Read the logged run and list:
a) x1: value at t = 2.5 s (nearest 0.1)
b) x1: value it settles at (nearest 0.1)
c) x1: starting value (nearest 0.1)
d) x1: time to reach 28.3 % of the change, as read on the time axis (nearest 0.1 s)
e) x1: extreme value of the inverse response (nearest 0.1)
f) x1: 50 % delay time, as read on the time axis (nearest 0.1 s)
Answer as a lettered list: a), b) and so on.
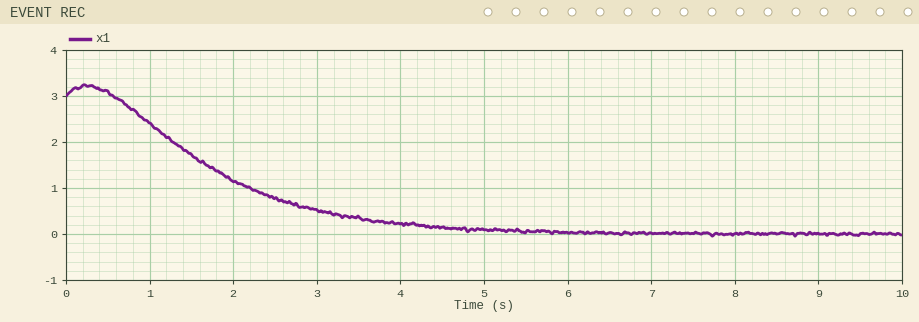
a) 0.8
b) 0.0
c) 3.0
d) 1.2 s
e) 3.2
f) 1.7 s
